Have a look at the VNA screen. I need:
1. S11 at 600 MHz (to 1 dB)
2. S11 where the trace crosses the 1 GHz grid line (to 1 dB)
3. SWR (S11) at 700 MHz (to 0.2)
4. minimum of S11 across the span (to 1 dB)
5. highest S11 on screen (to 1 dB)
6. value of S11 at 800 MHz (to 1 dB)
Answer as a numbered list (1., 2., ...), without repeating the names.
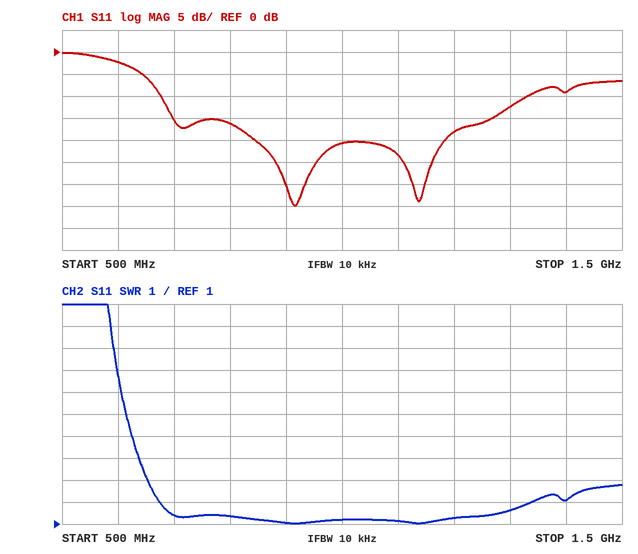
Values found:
1. -2 dB
2. -21 dB
3. 1.4
4. -35 dB
5. 0 dB
6. -16 dB
